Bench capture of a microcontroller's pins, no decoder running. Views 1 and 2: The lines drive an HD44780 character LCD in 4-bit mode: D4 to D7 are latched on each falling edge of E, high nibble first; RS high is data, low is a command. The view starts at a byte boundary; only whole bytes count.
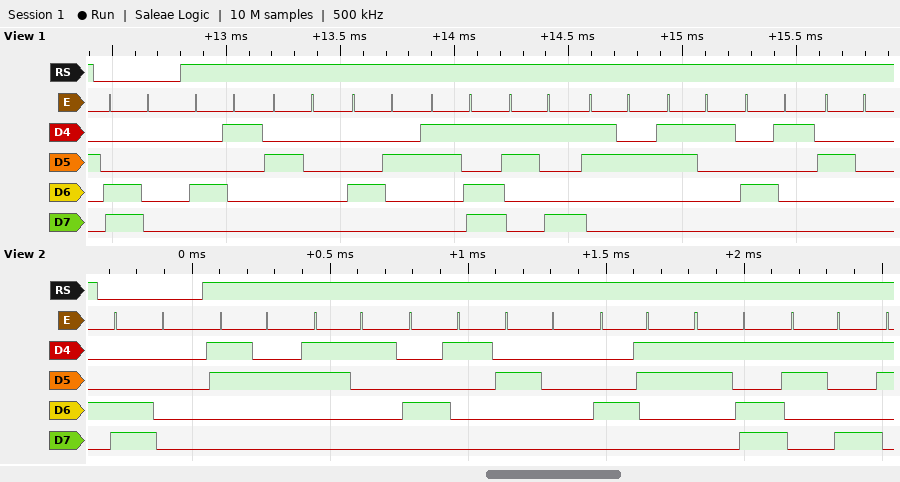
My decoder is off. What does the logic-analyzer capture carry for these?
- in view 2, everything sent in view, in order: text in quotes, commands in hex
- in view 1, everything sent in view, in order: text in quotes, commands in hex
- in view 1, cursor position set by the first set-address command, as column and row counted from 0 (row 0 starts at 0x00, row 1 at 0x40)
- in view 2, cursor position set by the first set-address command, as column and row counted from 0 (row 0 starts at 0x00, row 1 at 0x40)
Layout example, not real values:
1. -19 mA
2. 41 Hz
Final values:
1. 0xC0 "21A C=9"
2. 0xC0 "A B=921A "
3. column 0, row 1
4. column 0, row 1
